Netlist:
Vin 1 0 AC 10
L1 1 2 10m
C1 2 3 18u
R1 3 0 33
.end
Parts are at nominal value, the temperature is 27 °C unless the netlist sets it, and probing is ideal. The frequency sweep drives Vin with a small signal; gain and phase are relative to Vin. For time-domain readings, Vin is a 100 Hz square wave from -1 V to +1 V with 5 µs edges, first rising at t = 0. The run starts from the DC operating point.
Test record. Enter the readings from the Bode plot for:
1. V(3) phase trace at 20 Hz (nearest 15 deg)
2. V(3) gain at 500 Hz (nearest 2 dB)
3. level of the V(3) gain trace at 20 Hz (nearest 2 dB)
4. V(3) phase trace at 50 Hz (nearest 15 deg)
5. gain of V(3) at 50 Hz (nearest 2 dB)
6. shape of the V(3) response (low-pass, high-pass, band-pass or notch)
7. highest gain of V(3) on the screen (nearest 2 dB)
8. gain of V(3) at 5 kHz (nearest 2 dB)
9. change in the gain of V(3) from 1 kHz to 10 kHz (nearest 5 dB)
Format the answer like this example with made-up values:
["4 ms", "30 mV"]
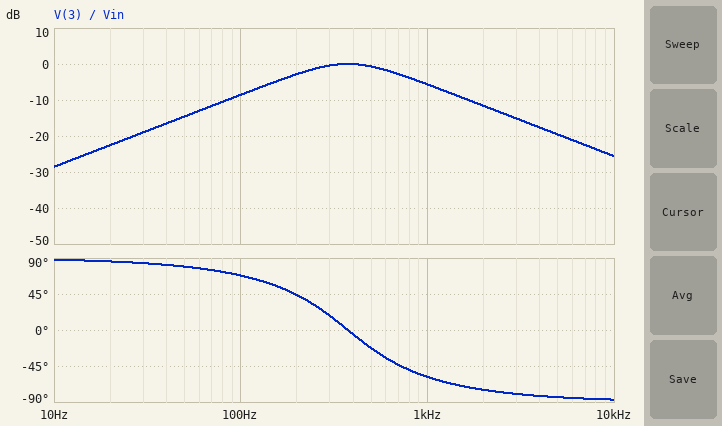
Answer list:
["90 deg", "0 dB", "-22 dB", "75 deg", "-14 dB", "band-pass", "0 dB", "-20 dB", "-20 dB"]
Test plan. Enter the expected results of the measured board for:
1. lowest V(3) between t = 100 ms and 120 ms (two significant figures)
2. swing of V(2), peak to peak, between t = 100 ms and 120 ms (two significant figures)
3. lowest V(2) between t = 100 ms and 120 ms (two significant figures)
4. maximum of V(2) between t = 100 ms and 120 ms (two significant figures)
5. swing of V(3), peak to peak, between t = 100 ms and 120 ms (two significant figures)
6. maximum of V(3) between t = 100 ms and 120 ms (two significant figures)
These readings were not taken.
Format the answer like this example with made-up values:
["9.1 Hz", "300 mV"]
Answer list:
["-1.3 V", "2.8 V", "-1.4 V", "1.4 V", "2.6 V", "1.3 V"]
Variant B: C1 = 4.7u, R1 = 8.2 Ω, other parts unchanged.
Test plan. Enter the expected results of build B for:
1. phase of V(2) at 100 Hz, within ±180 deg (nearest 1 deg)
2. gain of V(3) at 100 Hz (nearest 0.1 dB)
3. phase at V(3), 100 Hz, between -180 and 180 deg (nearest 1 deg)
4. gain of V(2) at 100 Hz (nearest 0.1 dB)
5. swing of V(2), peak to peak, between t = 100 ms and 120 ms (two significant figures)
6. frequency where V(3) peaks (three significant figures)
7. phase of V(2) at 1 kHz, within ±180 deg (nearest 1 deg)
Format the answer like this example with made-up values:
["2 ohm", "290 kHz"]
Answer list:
["0 deg", "-32.2 dB", "89 deg", "0.2 dB", "5.3 V", "734 Hz", "-151 deg"]
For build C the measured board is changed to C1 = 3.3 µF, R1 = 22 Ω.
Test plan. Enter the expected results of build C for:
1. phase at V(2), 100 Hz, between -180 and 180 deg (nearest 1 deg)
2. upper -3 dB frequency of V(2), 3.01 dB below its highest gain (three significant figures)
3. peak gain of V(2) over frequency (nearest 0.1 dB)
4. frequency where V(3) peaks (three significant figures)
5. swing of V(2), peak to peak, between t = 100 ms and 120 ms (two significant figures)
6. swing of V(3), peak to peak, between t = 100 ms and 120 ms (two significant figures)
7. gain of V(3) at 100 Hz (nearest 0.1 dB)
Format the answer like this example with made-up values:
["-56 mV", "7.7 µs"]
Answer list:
["0 deg", "1.01 kHz", "8.7 dB", "876 Hz", "4.3 V", "1.2 V", "-26.7 dB"]
